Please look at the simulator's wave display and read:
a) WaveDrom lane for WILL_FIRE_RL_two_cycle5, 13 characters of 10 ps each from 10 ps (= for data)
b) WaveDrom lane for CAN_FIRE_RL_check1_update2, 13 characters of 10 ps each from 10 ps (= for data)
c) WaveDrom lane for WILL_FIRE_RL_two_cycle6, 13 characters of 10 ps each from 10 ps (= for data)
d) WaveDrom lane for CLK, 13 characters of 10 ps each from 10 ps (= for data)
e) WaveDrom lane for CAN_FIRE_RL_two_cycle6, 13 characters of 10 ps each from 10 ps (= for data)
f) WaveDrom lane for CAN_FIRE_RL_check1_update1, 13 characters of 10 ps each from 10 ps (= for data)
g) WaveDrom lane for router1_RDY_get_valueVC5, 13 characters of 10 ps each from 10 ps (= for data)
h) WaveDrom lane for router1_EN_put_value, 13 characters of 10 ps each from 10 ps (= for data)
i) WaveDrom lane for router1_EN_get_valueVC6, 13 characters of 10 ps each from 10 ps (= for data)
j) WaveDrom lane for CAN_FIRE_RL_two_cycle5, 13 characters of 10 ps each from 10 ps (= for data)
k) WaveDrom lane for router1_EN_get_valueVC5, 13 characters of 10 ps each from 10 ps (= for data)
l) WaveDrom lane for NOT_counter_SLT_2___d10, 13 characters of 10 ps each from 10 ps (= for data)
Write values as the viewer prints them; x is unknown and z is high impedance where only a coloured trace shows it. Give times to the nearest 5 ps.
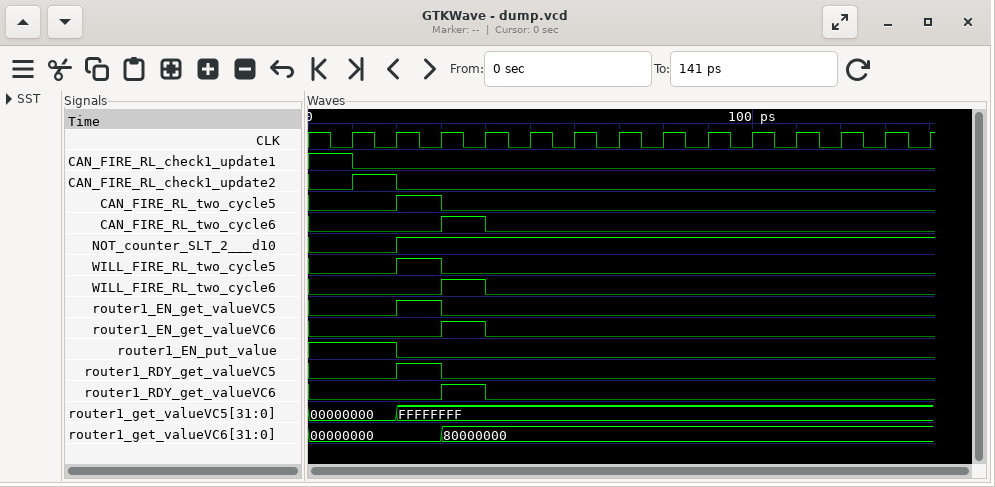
{name: 'WILL_FIRE_RL_two_cycle5', wave: '010..........'}
{name: 'CAN_FIRE_RL_check1_update2', wave: '10...........'}
{name: 'WILL_FIRE_RL_two_cycle6', wave: '0.10.........'}
{name: 'CLK', wave: 'p............'}
{name: 'CAN_FIRE_RL_two_cycle6', wave: '0.10.........'}
{name: 'CAN_FIRE_RL_check1_update1', wave: '0............'}
{name: 'router1_RDY_get_valueVC5', wave: '010..........'}
{name: 'router1_EN_put_value', wave: '10...........'}
{name: 'router1_EN_get_valueVC6', wave: '0.10.........'}
{name: 'CAN_FIRE_RL_two_cycle5', wave: '010..........'}
{name: 'router1_EN_get_valueVC5', wave: '010..........'}
{name: 'NOT_counter_SLT_2___d10', wave: '01...........'}
